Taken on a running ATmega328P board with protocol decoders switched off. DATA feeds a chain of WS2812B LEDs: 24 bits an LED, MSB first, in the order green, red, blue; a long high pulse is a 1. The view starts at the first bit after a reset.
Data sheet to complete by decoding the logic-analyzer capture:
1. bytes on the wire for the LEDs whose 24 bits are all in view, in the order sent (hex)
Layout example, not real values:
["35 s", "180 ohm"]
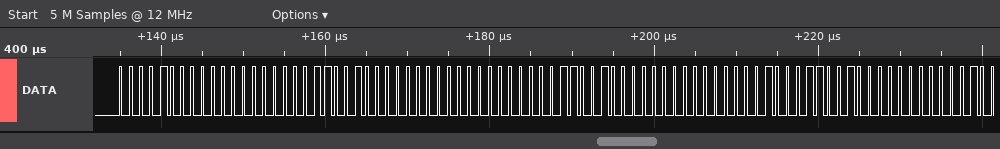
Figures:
["08 00 19 00 00 19 00 01 19"]
